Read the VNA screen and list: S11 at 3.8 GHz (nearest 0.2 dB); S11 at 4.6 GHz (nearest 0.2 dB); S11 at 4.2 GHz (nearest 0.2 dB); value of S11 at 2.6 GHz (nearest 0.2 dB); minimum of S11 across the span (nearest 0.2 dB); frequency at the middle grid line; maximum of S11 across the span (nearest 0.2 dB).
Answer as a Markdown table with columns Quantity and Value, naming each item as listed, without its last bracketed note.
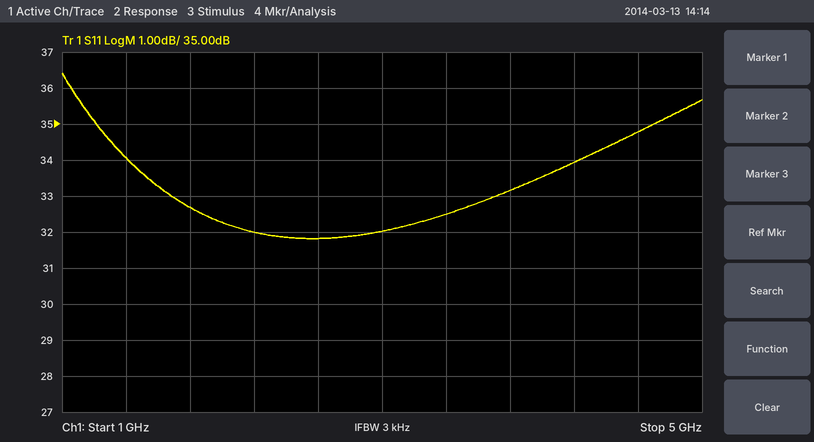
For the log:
| Quantity | Value |
|---|---|
| S11 at 3.8 GHz | 33.2 dB |
| S11 at 4.6 GHz | 34.8 dB |
| S11 at 4.2 GHz | 34.0 dB |
| value of S11 at 2.6 GHz | 31.8 dB |
| minimum of S11 across the span | 31.8 dB |
| frequency at the middle grid line | 3 GHz |
| maximum of S11 across the span | 36.4 dB |
